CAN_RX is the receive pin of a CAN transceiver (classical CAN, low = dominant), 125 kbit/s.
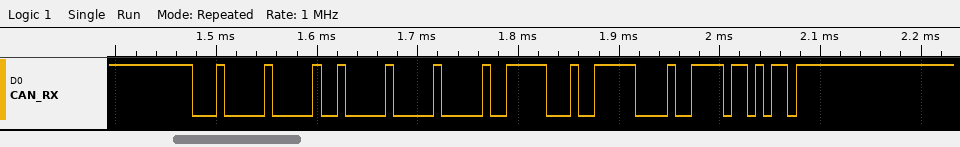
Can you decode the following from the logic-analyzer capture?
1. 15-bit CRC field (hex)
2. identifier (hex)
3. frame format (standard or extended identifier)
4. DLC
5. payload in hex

0x27B5
0x100
standard
4
00 01 F2 7C
